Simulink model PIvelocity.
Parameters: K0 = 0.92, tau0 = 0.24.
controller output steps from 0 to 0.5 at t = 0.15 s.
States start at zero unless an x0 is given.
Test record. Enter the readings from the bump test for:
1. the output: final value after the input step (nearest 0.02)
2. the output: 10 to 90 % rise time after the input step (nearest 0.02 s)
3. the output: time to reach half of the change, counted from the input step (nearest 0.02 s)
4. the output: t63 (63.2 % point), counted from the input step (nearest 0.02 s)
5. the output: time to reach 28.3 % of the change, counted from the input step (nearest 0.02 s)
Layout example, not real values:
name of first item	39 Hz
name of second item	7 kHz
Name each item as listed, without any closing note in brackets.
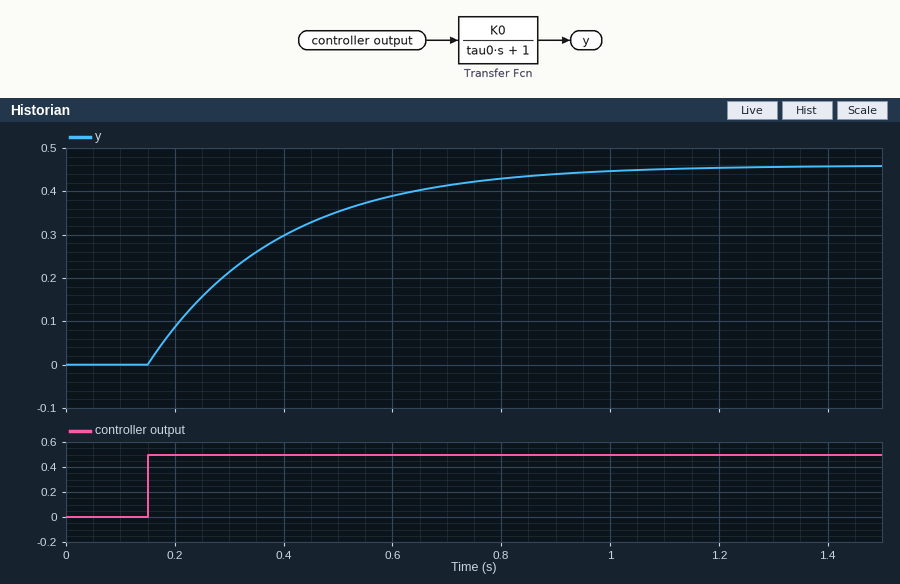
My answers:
the output: final value after the input step	0.46
the output: 10 to 90 % rise time after the input step	0.52 s
the output: time to reach half of the change, counted from the input step	0.16 s
the output: t63 (63.2 % point), counted from the input step	0.24 s
the output: time to reach 28.3 % of the change, counted from the input step	0.08 s
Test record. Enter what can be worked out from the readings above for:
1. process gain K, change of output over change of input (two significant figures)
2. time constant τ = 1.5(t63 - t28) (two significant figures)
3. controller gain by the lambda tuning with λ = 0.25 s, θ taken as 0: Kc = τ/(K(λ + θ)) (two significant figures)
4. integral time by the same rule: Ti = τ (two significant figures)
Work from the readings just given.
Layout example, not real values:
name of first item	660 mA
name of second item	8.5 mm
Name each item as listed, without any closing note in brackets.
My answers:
process gain K, change of output over change of input	0.92
time constant τ = 1.5(t63 - t28)	0.24 s
controller gain by the lambda tuning with λ = 0.25 s, θ taken as 0: Kc = τ/(K(λ + θ))	1.0
integral time by the same rule: Ti = τ	0.24 s
